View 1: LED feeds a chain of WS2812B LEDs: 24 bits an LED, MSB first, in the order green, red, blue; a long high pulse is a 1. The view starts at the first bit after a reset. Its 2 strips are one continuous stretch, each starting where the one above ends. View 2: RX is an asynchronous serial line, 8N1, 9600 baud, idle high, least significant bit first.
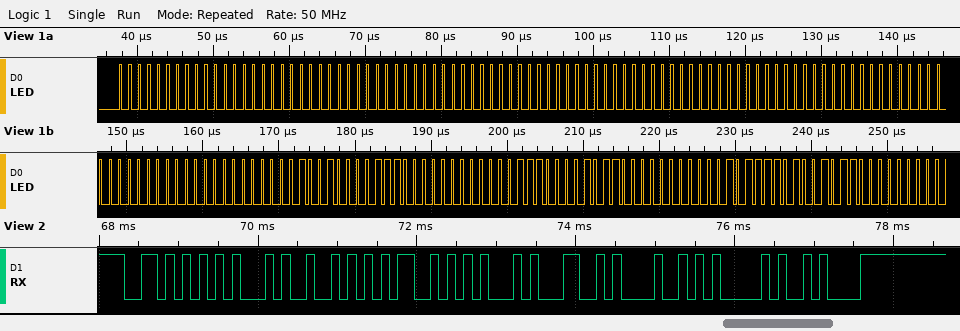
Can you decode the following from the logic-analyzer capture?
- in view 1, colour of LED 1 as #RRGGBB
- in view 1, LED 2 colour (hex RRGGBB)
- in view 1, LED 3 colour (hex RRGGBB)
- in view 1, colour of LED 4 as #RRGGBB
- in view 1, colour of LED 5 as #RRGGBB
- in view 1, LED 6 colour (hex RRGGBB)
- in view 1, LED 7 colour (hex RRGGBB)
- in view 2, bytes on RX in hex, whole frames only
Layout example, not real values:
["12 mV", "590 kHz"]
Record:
["#000000", "#000000", "#000000", "#000000", "#09000E", "#1C002C", "#5E0096", "0x56 0x45 0x52 0x4D 0x45 0x4C 0x48 0x41 0x0A"]
